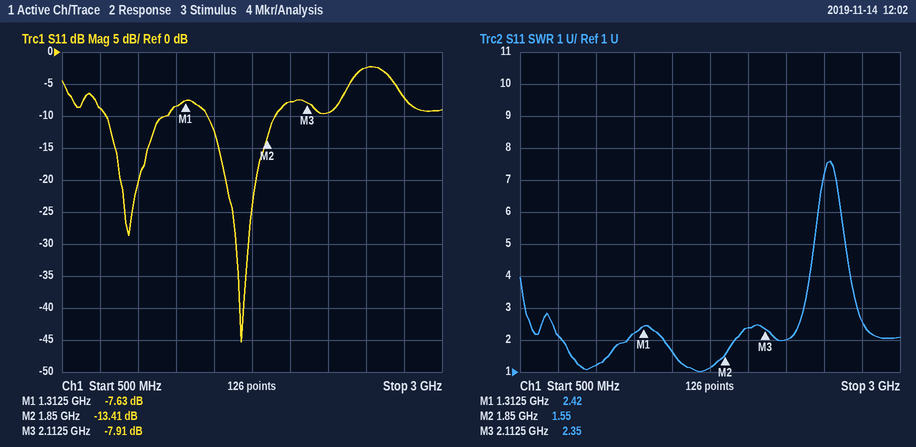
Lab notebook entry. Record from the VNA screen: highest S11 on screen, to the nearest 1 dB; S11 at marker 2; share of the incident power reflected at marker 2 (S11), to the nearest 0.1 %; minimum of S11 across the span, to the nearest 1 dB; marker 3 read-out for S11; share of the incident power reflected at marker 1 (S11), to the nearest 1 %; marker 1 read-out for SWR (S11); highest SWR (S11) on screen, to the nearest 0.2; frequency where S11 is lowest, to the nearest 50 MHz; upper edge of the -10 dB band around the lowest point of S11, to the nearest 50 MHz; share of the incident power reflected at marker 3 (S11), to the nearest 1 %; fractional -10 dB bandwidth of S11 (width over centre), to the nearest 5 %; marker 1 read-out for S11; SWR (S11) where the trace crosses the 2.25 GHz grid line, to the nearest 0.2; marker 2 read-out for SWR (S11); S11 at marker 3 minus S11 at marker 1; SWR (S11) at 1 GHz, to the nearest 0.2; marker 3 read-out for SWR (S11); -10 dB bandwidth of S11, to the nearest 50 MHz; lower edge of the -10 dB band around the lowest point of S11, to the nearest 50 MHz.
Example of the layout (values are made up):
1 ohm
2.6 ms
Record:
-2 dB
-13.41 dB
4.6 %
-45 dB
-7.91 dB
17 %
2.42
7.6
1.70 GHz
1.90 GHz
16 %
25 %
-7.63 dB
2.0
1.55
-0.28 dB
1.2
2.35
450 MHz
1.45 GHz
